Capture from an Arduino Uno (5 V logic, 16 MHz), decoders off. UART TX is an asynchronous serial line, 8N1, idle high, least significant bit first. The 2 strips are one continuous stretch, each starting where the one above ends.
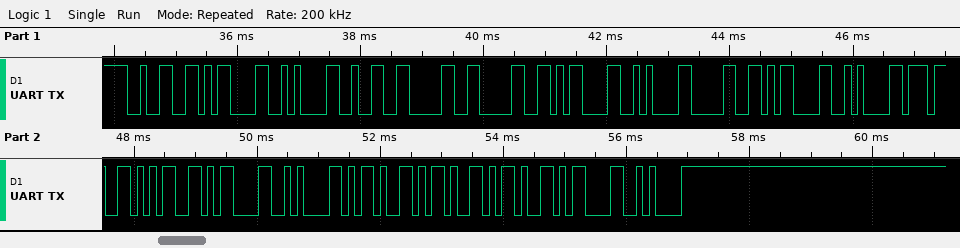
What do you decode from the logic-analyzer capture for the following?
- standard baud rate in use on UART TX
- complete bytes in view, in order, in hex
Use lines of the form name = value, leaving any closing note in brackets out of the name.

standard baud rate in use on UART TX = 9600 baud
complete bytes in view, in order, in hex = 32 0D 0A 32 30 30 0D 0A 30 0D 0A 37 35 0D 0A 2D 2D 2D 0D 0A
